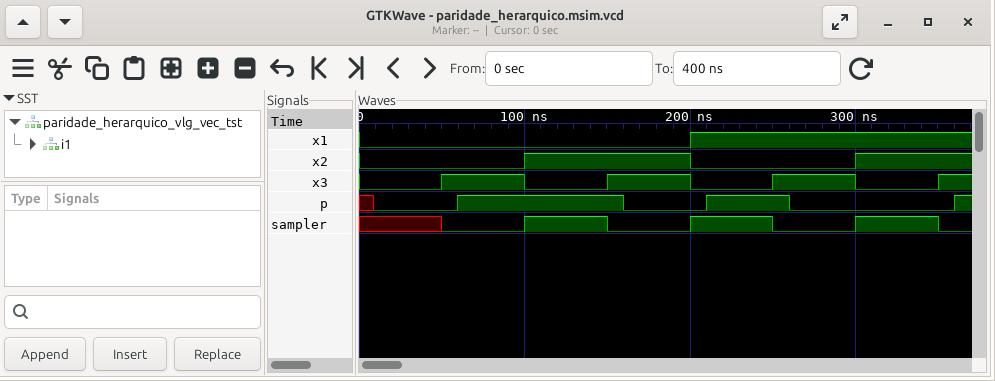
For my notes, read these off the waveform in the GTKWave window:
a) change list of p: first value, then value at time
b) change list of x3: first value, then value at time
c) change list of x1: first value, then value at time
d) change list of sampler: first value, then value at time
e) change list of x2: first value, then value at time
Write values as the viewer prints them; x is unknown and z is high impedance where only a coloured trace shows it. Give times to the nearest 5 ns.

x, 0 at 10 ns, 1 at 60 ns, 0 at 160 ns, 1 at 210 ns, 0 at 260 ns, 1 at 360 ns
0, 1 at 50 ns, 0 at 100 ns, 1 at 150 ns, 0 at 200 ns, 1 at 250 ns, 0 at 300 ns, 1 at 350 ns
0, 1 at 200 ns
x, 0 at 50 ns, 1 at 100 ns, 0 at 150 ns, 1 at 200 ns, 0 at 250 ns, 1 at 300 ns, 0 at 350 ns
0, 1 at 100 ns, 0 at 200 ns, 1 at 300 ns
